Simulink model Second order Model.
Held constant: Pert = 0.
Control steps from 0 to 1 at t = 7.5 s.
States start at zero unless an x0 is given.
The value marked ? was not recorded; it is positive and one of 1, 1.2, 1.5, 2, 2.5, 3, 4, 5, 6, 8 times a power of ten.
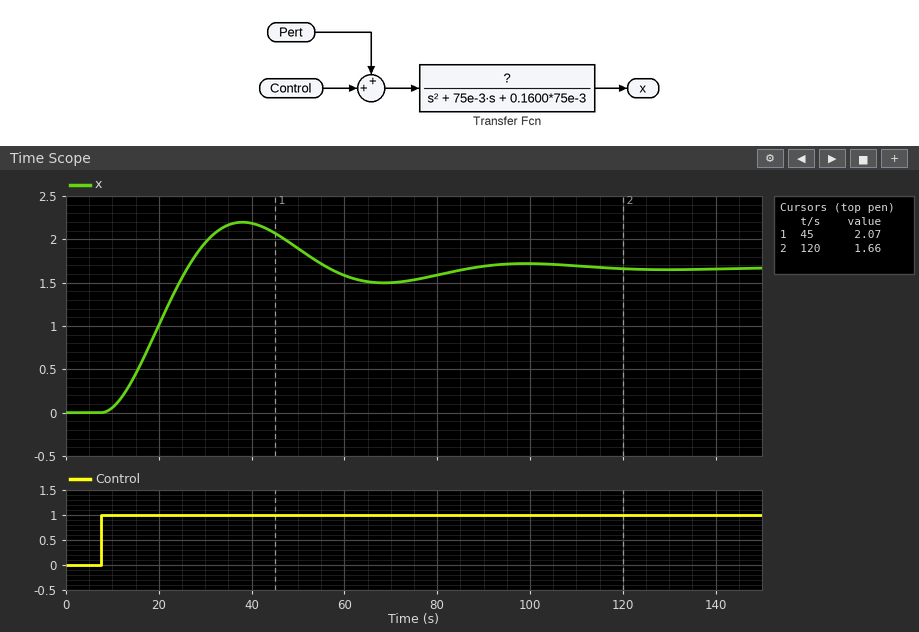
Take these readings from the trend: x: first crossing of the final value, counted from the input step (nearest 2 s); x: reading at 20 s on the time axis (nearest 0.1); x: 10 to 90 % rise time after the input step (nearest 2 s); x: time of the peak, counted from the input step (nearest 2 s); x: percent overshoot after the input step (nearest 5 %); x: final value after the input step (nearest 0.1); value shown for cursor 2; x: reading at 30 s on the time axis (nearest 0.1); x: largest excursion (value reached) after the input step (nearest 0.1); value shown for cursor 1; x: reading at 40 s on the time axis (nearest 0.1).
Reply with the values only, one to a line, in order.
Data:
18 s
1.0
12 s
30 s
30 %
1.7
1.66
2.0
2.2
2.07
2.2
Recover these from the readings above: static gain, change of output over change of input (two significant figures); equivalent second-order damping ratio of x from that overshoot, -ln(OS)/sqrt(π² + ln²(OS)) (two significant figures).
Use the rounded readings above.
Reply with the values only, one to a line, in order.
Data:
1.7
0.36
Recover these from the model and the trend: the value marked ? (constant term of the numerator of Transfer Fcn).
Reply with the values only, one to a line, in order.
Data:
0.02
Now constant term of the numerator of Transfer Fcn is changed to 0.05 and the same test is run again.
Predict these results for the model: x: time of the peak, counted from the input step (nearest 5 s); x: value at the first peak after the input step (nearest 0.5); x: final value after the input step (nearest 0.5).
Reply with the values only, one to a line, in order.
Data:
30 s
5.5
4.0
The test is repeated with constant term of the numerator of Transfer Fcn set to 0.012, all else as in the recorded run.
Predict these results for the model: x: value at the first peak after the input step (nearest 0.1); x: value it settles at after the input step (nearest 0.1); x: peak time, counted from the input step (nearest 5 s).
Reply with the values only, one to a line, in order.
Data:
1.3
1.0
30 s
